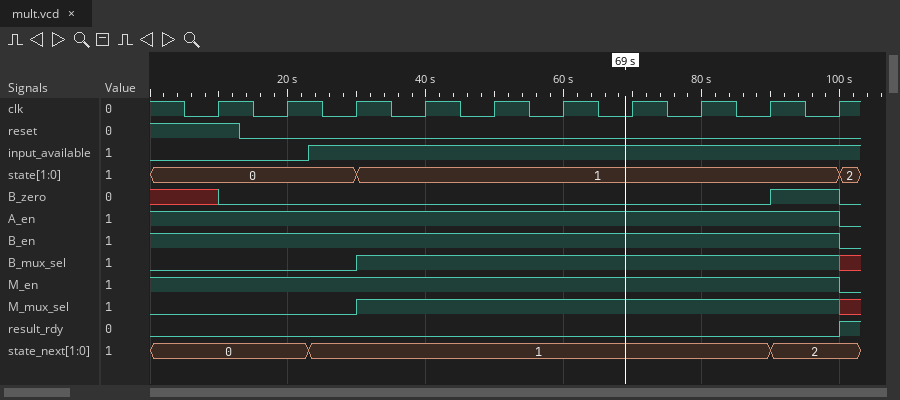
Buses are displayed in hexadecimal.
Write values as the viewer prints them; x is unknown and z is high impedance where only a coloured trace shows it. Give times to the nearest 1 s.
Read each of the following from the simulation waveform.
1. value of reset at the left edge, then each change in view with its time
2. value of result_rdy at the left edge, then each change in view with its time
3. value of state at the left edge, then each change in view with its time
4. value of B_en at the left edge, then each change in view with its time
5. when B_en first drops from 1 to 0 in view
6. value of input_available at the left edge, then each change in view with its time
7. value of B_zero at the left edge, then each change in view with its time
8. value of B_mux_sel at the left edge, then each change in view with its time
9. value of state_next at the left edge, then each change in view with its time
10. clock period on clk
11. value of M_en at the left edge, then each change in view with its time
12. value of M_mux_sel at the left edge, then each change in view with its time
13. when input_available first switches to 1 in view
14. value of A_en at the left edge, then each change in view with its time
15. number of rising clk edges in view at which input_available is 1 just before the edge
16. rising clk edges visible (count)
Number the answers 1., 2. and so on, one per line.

1. 1, 0 at 13 s
2. 0, 1 at 100 s
3. 0, 1 at 30 s, 2 at 100 s
4. 1, 0 at 100 s
5. 100 s
6. 0, 1 at 23 s
7. x, 0 at 10 s, 1 at 90 s, 0 at 100 s
8. 0, 1 at 30 s, x at 100 s
9. 0, 1 at 23 s, 2 at 90 s
10. 10 s
11. 1, 0 at 100 s
12. 0, 1 at 30 s, x at 100 s
13. 23 s
14. 1, 0 at 100 s
15. 8
16. 10
